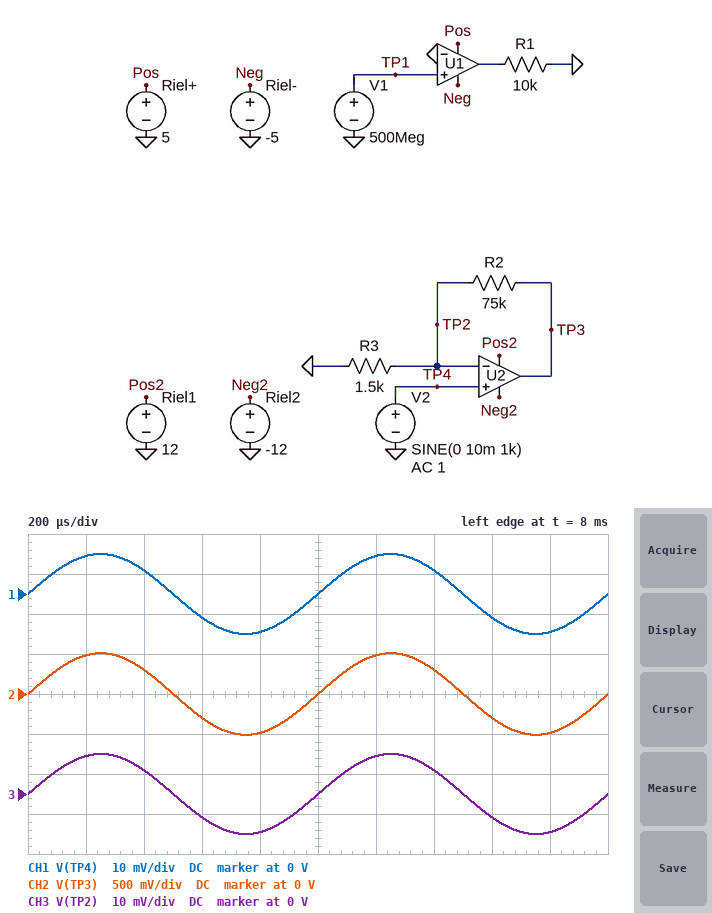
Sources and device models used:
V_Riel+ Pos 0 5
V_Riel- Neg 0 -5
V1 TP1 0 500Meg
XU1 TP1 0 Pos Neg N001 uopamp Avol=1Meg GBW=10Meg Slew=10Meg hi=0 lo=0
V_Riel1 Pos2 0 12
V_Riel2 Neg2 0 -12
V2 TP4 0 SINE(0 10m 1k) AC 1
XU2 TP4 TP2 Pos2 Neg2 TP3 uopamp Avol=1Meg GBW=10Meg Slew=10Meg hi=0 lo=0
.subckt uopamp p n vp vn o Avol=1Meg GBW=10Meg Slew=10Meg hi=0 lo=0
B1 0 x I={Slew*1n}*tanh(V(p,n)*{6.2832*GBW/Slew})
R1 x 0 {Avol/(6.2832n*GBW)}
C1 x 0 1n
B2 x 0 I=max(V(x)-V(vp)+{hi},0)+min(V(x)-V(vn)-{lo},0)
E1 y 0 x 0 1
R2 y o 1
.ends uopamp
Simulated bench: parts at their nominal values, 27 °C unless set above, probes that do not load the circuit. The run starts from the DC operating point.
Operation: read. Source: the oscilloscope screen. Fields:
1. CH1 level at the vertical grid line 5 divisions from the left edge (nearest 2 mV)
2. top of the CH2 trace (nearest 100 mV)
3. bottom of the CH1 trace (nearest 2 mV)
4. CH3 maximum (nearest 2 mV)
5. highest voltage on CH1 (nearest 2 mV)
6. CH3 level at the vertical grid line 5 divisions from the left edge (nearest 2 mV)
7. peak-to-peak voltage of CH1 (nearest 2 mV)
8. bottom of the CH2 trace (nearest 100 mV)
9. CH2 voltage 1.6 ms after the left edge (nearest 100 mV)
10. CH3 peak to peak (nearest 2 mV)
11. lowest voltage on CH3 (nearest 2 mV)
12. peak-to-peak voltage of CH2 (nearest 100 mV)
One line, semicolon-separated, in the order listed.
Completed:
0 V; 500 mV; -10 mV; 10 mV; 10 mV; 0 V; 20 mV; -500 mV; -300 mV; 20 mV; -10 mV; 1.0 V
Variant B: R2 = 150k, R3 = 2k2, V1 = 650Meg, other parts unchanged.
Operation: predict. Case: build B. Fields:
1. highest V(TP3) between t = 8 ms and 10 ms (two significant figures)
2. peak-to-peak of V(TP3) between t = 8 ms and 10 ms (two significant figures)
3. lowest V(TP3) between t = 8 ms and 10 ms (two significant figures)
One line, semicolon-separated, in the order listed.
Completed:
690 mV; 1.4 V; -690 mV
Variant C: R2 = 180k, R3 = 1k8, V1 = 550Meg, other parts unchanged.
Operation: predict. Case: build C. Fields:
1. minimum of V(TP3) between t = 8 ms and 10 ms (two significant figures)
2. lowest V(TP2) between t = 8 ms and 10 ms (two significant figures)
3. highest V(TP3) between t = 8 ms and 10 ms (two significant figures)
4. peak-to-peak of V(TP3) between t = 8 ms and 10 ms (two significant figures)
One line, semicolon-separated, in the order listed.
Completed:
-1.0 V; -10 mV; 1.0 V; 2.0 V
